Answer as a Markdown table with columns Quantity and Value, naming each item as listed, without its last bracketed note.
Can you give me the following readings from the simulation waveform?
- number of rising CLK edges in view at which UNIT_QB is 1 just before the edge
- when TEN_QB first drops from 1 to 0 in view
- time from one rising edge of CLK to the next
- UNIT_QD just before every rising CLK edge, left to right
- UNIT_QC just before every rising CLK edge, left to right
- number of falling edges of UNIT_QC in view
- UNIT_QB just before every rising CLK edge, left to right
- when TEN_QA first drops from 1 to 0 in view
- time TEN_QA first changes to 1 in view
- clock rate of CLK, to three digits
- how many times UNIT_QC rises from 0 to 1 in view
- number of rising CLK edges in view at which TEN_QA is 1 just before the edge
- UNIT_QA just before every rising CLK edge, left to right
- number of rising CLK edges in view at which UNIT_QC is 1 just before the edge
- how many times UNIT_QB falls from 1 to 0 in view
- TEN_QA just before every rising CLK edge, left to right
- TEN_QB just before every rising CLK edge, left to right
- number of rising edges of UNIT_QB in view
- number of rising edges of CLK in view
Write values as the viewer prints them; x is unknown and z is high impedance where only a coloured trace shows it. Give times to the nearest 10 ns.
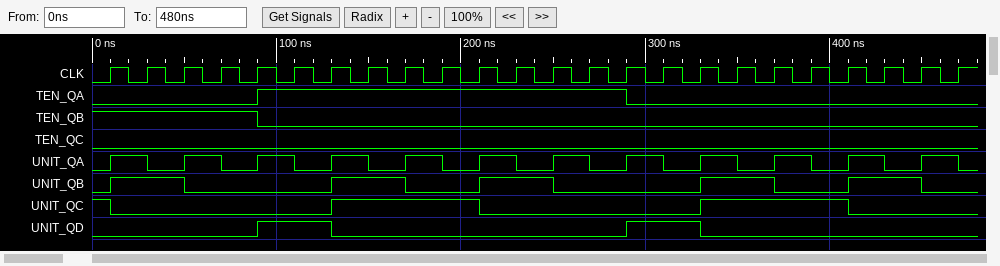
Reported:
| Quantity | Value |
|---|---|
| number of rising CLK edges in view at which UNIT_QB is 1 just before the edge | 10 |
| when TEN_QB first drops from 1 to 0 in view | 90 ns |
| time from one rising edge of CLK to the next | 20 ns |
| UNIT_QD just before every rising CLK edge, left to right | 0 0 0 0 0 1 1 0 0 0 0 0 0 0 0 1 1 0 0 0 0 0 0 0 |
| UNIT_QC just before every rising CLK edge, left to right | 1 0 0 0 0 0 0 1 1 1 1 0 0 0 0 0 0 1 1 1 1 0 0 0 |
| number of falling edges of UNIT_QC in view | 3 |
| UNIT_QB just before every rising CLK edge, left to right | 0 1 1 0 0 0 0 1 1 0 0 1 1 0 0 0 0 1 1 0 0 1 1 0 |
| when TEN_QA first drops from 1 to 0 in view | 290 ns |
| time TEN_QA first changes to 1 in view | 90 ns |
| clock rate of CLK, to three digits | 50.0 MHz |
| how many times UNIT_QC rises from 0 to 1 in view | 2 |
| number of rising CLK edges in view at which TEN_QA is 1 just before the edge | 10 |
| UNIT_QA just before every rising CLK edge, left to right | 0 1 0 1 0 1 0 1 0 1 0 1 0 1 0 1 0 1 0 1 0 1 0 1 |
| number of rising CLK edges in view at which UNIT_QC is 1 just before the edge | 9 |
| how many times UNIT_QB falls from 1 to 0 in view | 5 |
| TEN_QA just before every rising CLK edge, left to right | 0 0 0 0 0 1 1 1 1 1 1 1 1 1 1 0 0 0 0 0 0 0 0 0 |
| TEN_QB just before every rising CLK edge, left to right | 1 1 1 1 1 0 0 0 0 0 0 0 0 0 0 0 0 0 0 0 0 0 0 0 |
| number of rising edges of UNIT_QB in view | 5 |
| number of rising edges of CLK in view | 24 |
